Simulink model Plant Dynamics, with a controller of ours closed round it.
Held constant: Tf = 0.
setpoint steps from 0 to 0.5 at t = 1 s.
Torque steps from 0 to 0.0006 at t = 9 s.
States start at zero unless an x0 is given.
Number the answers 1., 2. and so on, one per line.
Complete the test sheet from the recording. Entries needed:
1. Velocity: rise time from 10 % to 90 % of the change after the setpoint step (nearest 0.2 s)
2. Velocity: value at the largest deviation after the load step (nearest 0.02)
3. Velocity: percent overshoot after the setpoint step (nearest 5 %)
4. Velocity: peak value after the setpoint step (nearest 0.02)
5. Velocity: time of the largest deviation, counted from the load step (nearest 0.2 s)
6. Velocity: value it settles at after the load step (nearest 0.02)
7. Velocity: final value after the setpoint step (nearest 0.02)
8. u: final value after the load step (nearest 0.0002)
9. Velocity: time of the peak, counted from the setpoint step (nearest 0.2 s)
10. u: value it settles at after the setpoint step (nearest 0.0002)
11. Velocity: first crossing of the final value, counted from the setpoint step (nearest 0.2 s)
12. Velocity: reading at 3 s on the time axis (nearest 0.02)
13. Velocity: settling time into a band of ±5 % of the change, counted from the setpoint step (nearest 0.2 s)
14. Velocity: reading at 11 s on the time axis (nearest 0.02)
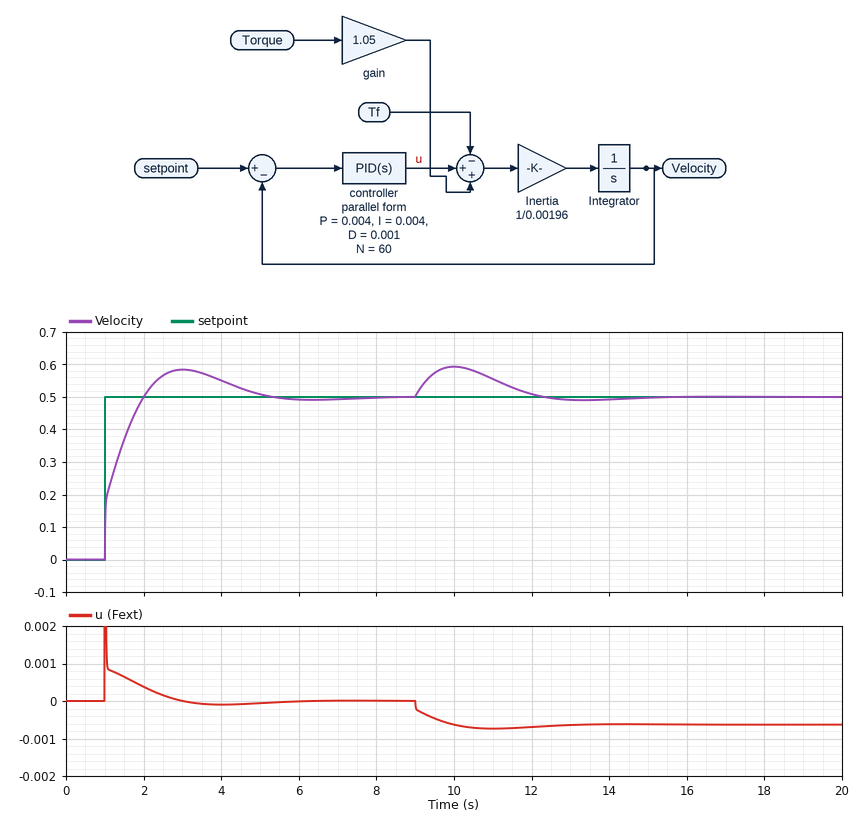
1. 0.8 s
2. 0.60
3. 15 %
4. 0.58
5. 1.0 s
6. 0.50
7. 0.50
8. -0.0006
9. 2.0 s
10. 0.0000
11. 1.0 s
12. 0.58
13. 3.6 s
14. 0.56
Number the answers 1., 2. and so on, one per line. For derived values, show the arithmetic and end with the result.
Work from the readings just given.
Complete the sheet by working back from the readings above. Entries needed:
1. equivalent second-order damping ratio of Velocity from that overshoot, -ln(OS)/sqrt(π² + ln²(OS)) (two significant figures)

1. ln(0.15) = -1.897; 1.897 / sqrt(9.870 + 3.599) = 0.52
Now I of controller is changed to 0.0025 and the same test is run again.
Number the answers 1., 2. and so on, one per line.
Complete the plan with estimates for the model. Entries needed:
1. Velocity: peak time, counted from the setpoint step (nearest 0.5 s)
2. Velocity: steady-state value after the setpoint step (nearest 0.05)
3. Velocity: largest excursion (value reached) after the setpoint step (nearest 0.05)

1. 2.5 s
2. 0.50
3. 0.55
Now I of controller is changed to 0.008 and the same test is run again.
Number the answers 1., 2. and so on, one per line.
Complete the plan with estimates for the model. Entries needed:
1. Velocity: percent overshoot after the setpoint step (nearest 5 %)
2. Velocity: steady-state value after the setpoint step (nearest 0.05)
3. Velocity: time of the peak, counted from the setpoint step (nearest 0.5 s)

1. 25 %
2. 0.50
3. 1.5 s
